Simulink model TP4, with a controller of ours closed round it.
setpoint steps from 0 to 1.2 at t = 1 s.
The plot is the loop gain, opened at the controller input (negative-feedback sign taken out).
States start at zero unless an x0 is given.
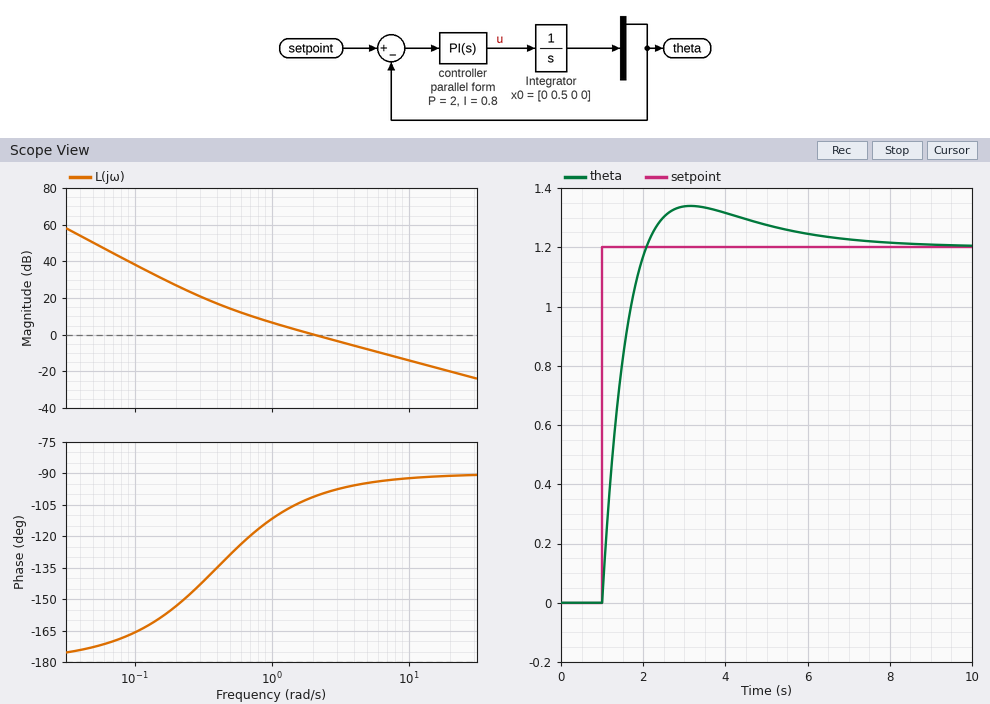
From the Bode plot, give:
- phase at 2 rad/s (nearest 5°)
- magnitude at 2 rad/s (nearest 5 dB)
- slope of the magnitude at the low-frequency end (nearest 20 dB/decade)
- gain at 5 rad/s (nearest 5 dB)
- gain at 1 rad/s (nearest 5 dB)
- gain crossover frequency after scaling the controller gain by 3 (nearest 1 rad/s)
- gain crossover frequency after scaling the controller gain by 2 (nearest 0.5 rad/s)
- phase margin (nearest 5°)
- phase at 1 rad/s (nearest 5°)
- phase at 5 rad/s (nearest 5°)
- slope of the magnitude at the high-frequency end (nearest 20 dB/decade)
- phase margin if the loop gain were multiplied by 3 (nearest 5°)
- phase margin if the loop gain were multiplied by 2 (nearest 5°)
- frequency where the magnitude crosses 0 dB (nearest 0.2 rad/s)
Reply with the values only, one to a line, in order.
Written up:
-100°
0 dB
-40 dB/decade
-10 dB
5 dB
6 rad/s
4.0 rad/s
80°
-110°
-95°
-20 dB/decade
85°
85°
2.0 rad/s
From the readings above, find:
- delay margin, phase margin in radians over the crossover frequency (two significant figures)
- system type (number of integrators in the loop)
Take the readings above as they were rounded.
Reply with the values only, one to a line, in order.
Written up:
0.70 s
2
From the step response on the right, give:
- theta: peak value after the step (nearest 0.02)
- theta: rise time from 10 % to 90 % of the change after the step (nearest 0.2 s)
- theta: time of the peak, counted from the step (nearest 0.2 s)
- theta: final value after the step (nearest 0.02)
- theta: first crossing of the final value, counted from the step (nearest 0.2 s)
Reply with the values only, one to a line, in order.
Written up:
1.34
0.8 s
2.2 s
1.20
1.0 s
